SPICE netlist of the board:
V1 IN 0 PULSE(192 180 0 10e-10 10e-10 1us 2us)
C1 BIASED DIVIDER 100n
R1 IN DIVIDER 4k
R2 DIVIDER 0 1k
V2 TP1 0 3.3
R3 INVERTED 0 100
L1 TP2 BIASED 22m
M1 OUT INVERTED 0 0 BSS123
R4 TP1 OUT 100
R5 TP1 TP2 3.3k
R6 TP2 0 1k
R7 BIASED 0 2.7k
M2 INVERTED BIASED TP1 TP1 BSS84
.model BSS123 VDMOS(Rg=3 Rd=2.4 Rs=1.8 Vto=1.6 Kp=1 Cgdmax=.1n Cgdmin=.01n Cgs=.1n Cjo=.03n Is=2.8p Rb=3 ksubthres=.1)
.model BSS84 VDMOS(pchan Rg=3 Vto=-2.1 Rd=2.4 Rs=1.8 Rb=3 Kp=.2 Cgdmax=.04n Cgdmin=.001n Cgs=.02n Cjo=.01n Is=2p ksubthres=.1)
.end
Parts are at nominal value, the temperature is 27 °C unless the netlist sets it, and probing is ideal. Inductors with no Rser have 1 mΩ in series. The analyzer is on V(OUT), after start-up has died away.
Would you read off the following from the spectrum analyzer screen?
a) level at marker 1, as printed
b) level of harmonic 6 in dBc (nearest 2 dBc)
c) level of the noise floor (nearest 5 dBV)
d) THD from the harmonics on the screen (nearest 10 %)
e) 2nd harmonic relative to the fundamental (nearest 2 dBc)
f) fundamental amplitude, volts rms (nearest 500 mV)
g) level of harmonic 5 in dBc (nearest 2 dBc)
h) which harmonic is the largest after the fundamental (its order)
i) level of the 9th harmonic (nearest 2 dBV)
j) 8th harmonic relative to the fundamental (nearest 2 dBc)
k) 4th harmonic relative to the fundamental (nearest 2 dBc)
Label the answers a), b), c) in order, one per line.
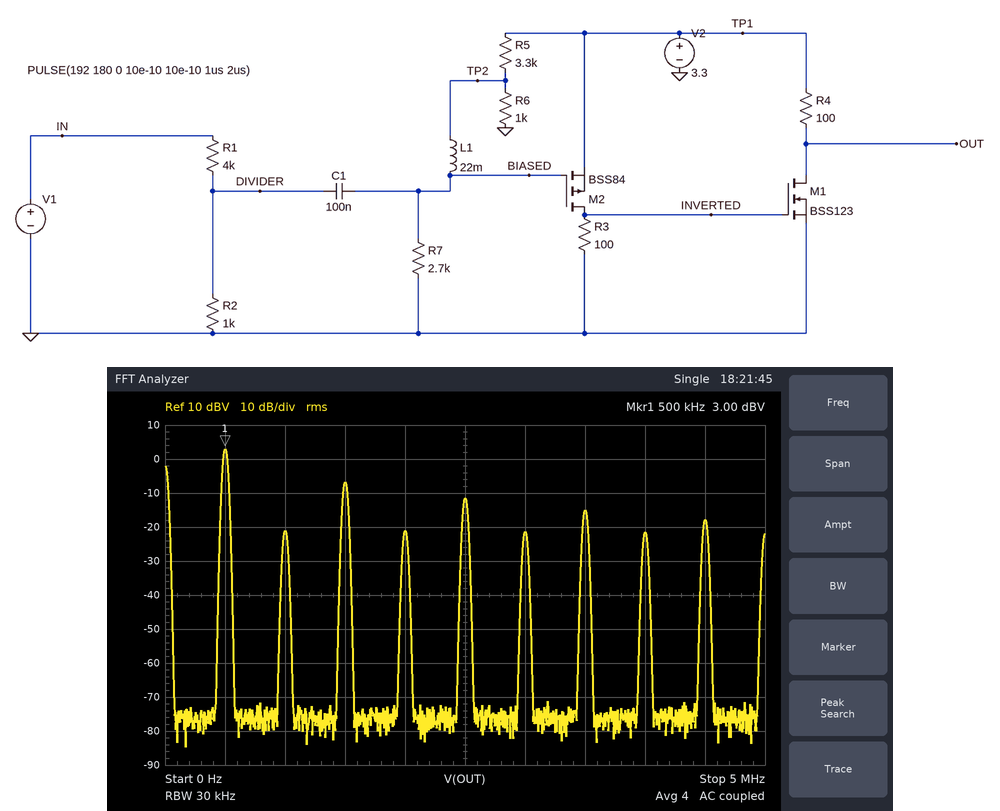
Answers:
a) 3.00 dBV
b) -24 dBc
c) -75 dBV
d) 40 %
e) -24 dBc
f) 1.5 V
g) -14 dBc
h) 3
i) -18 dBV
j) -24 dBc
k) -24 dBc
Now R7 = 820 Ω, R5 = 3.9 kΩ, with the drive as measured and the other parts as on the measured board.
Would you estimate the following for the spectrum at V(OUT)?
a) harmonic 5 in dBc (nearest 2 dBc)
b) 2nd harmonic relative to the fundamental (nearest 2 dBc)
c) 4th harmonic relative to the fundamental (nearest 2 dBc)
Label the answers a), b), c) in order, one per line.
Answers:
a) -18 dBc
b) -14 dBc
c) -16 dBc
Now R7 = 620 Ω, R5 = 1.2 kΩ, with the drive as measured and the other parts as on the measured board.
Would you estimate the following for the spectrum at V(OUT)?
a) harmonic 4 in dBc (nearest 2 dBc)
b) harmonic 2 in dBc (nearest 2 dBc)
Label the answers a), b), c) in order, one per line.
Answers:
a) -42 dBc
b) -42 dBc
